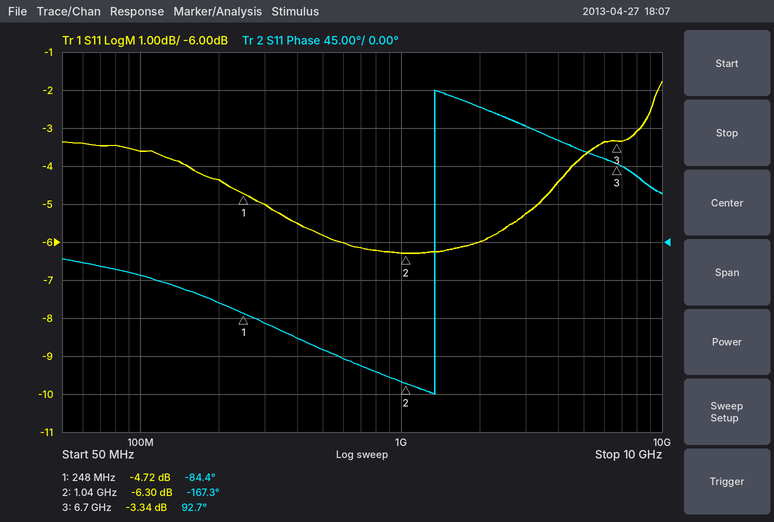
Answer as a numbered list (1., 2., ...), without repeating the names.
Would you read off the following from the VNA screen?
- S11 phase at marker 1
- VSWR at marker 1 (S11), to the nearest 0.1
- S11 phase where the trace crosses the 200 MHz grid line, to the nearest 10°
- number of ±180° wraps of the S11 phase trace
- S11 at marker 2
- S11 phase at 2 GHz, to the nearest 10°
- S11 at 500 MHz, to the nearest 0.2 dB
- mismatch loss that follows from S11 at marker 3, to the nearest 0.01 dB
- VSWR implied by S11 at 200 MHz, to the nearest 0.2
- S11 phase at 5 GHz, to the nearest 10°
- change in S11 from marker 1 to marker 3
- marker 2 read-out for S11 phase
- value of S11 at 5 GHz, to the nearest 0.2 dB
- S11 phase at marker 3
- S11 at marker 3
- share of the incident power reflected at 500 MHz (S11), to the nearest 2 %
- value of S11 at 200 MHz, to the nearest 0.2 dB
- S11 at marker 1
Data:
1. -84.4°
2. 3.8
3. -70°
4. 1
5. -6.30 dB
6. 160°
7. -5.8 dB
8. 2.70 dB
9. 4.0
10. 110°
11. 1.38 dB
12. -167.3°
13. -3.8 dB
14. 92.7°
15. -3.34 dB
16. 26 %
17. -4.4 dB
18. -4.72 dB
